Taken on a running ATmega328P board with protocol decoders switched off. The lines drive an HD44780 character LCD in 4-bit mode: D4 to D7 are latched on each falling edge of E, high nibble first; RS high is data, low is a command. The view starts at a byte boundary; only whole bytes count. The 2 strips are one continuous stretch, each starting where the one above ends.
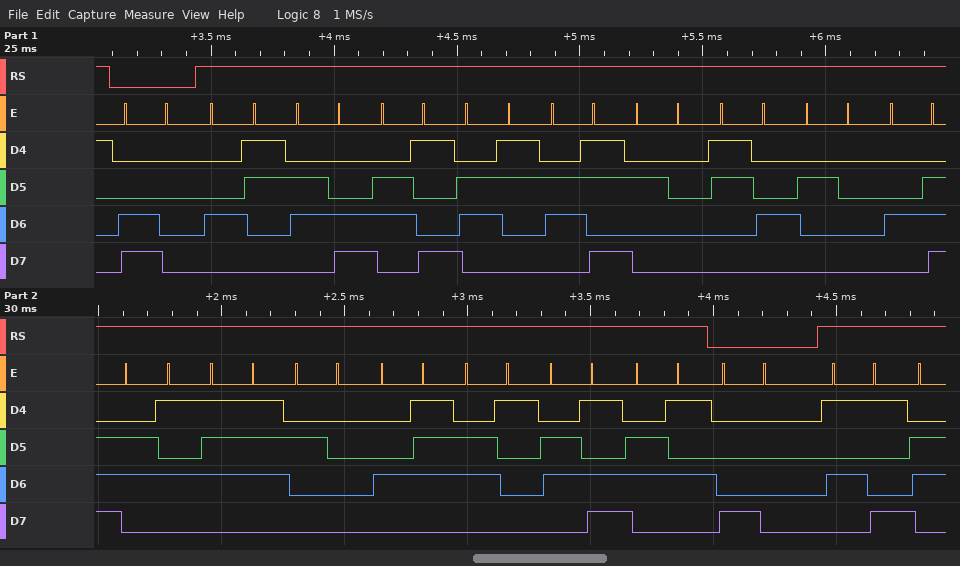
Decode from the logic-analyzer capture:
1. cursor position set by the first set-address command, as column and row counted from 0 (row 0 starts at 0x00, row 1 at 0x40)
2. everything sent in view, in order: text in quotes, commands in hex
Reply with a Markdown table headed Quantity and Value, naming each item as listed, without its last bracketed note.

| Quantity | Value |
|---|---|
| cursor position set by the first set-address command, as column and row counted from 0 | column 0, row 1 |
| everything sent in view, in order: text in quotes, commands in hex | 0xC0 "Click 4 New Game" 0x80 "Y" |
